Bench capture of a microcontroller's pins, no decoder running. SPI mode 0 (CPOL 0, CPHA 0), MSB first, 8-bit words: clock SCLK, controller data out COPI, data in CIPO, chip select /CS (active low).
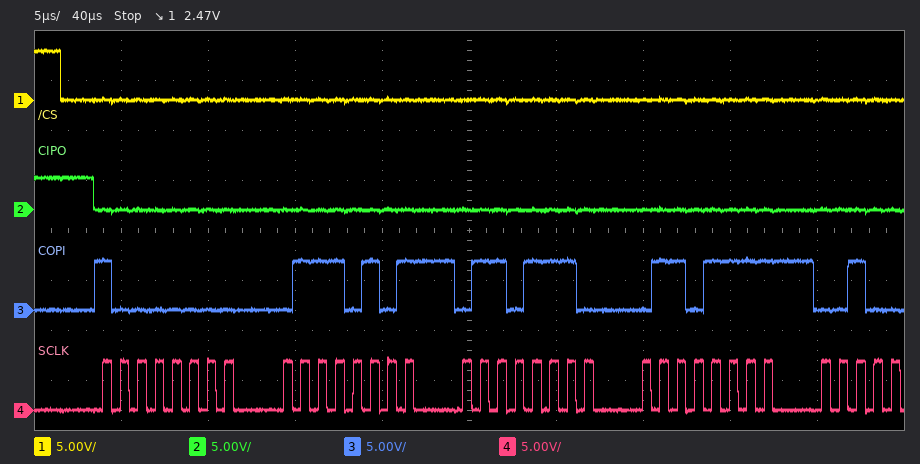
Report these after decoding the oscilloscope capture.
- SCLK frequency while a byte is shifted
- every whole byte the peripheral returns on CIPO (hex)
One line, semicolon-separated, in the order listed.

1 MHz; 00 00 00 00
